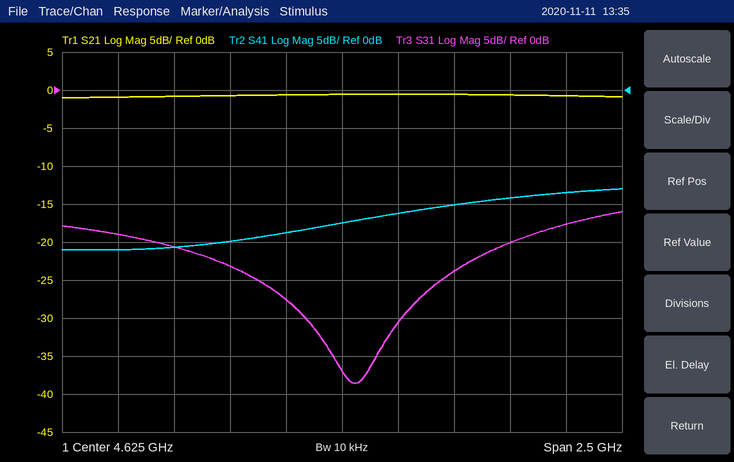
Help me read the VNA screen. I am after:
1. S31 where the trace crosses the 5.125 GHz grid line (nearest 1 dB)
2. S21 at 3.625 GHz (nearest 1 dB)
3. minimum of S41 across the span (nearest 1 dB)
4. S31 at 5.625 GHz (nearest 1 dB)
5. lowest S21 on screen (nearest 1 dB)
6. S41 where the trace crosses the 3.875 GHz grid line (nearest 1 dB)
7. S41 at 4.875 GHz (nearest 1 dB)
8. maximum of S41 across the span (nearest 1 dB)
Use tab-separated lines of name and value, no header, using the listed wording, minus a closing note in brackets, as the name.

S31 where the trace crosses the 5.125 GHz grid line	-24 dB
S21 at 3.625 GHz	-1 dB
minimum of S41 across the span	-21 dB
S31 at 5.625 GHz	-18 dB
lowest S21 on screen	-1 dB
S41 where the trace crosses the 3.875 GHz grid line	-21 dB
S41 at 4.875 GHz	-16 dB
maximum of S41 across the span	-13 dB
